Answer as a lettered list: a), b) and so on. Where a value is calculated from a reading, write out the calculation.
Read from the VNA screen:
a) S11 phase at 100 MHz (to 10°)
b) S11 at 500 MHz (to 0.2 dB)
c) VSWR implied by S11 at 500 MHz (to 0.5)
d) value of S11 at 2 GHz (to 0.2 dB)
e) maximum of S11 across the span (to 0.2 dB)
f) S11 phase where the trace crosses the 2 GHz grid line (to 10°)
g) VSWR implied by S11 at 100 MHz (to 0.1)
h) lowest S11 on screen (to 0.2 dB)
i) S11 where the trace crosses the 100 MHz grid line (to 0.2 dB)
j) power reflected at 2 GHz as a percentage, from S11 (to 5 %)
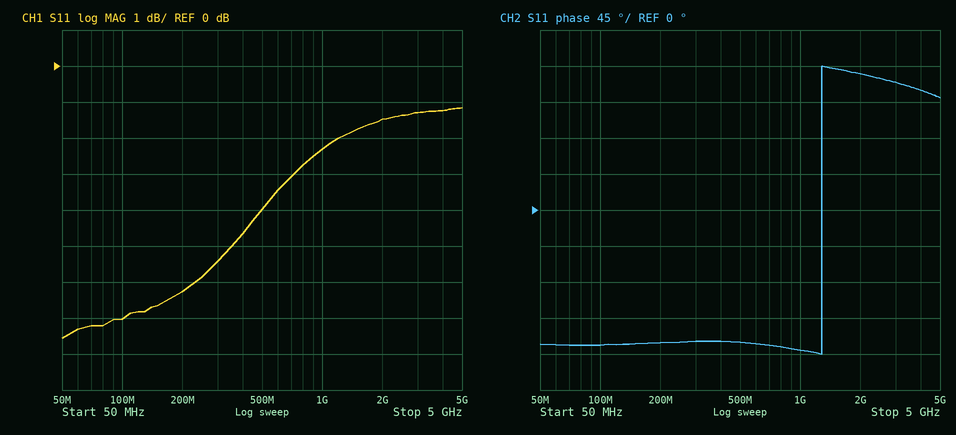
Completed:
a) -170°
b) -4.0 dB
c) |Γ| = 10^(-4/20) = 0.6310; VSWR = (1 + 0.6310)/(1 − 0.6310) ≈ 4.42, so 4.5 to the nearest 0.5
d) -1.4 dB
e) -1.2 dB
f) 170°
g) |Γ| = 10^(-7/20) = 0.4467; VSWR = (1 + 0.4467)/(1 − 0.4467) ≈ 2.6
h) -7.6 dB
i) -7.0 dB
j) 10^(-1.4/10) ≈ 72.4 %, so 70 % to the nearest 5 %
